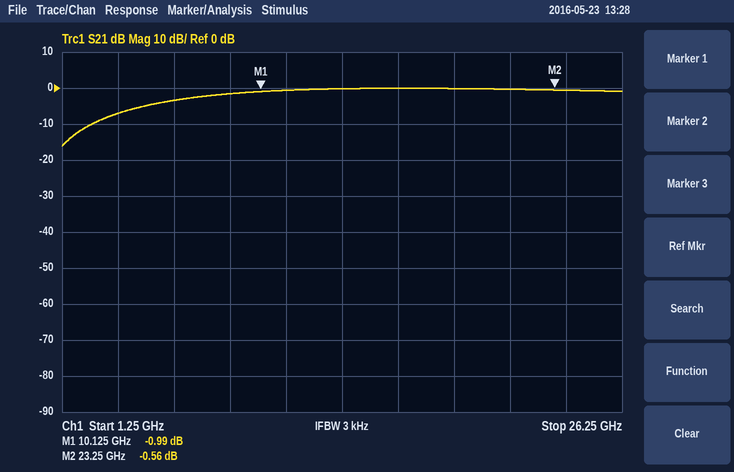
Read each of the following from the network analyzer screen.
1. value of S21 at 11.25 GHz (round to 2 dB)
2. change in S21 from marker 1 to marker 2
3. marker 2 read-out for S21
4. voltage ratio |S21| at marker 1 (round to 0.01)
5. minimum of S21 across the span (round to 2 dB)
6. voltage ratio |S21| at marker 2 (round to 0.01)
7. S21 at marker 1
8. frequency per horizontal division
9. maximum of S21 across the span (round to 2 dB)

0 dB
0.43 dB
-0.56 dB
0.89
-16 dB
0.94
-0.99 dB
2.5 GHz
0 dB
